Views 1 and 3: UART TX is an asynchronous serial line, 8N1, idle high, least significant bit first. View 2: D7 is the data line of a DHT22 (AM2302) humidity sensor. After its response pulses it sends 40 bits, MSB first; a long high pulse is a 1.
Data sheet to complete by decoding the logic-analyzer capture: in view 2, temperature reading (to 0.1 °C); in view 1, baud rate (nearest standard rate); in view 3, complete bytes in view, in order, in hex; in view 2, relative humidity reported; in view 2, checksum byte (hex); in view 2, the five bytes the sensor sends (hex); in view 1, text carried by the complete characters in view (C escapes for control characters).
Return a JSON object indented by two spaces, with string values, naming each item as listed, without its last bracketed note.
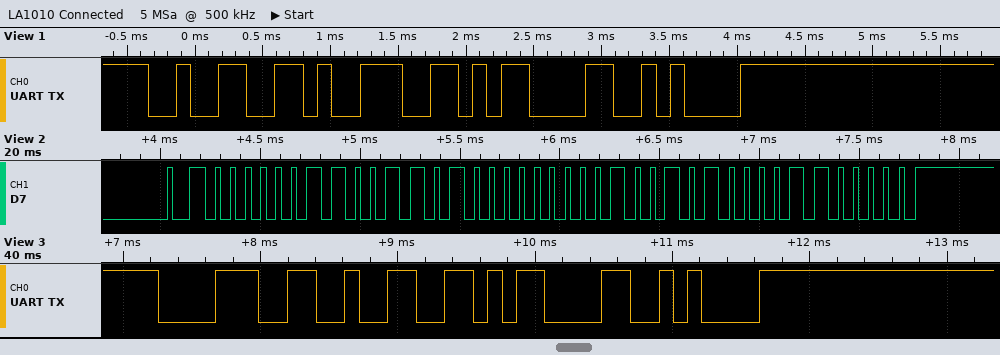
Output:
{
  "in view 2, temperature reading": "29.6 °C",
  "in view 1, baud rate": "9600 baud",
  "in view 3, complete bytes in view, in order, in hex": "38 32 0D 0A",
  "in view 2, relative humidity reported": "82.0 %",
  "in view 2, checksum byte": "0x60",
  "in view 2, the five bytes the sensor sends": "03 34 01 28 60",
  "in view 1, text carried by the complete characters in view": "\"29\\r\\n\""
}
